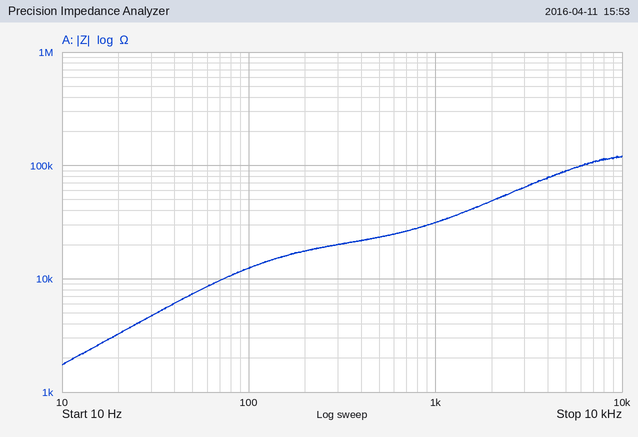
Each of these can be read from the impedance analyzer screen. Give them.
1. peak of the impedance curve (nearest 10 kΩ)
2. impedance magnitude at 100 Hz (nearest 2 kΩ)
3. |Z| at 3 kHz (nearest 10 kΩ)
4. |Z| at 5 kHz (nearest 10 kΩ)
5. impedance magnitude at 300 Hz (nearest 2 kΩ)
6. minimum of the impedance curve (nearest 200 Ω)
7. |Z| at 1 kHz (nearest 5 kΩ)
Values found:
120 kΩ
12 kΩ
60 kΩ
90 kΩ
20 kΩ
1.8 kΩ
30 kΩ
